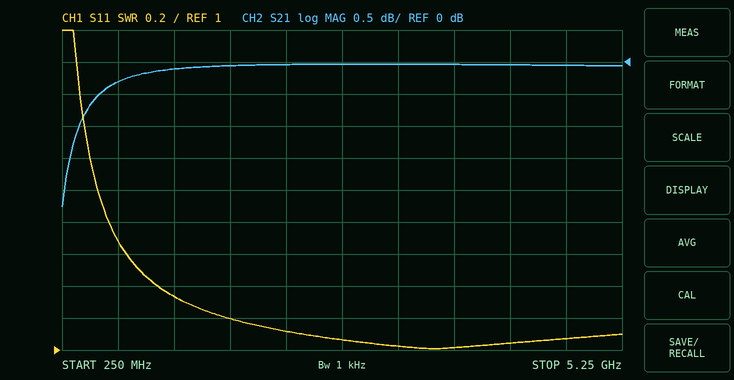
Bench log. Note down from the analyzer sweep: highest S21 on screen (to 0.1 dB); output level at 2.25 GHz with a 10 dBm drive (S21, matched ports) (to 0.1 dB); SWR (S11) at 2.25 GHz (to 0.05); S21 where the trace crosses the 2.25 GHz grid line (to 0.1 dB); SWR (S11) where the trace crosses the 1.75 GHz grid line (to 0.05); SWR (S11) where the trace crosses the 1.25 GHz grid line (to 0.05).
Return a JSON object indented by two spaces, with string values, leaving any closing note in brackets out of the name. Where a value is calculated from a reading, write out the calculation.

{
  "highest S21 on screen": "0.0 dB",
  "output level at 2.25 GHz with a 10 dBm drive (S21, matched ports)": "10 dBm + (0.0 dB) = 10.0 dBm",
  "SWR (S11) at 2.25 GHz": "1.10",
  "S21 where the trace crosses the 2.25 GHz grid line": "0.0 dB",
  "SWR (S11) where the trace crosses the 1.75 GHz grid line": "1.20",
  "SWR (S11) where the trace crosses the 1.25 GHz grid line": "1.35"
}
